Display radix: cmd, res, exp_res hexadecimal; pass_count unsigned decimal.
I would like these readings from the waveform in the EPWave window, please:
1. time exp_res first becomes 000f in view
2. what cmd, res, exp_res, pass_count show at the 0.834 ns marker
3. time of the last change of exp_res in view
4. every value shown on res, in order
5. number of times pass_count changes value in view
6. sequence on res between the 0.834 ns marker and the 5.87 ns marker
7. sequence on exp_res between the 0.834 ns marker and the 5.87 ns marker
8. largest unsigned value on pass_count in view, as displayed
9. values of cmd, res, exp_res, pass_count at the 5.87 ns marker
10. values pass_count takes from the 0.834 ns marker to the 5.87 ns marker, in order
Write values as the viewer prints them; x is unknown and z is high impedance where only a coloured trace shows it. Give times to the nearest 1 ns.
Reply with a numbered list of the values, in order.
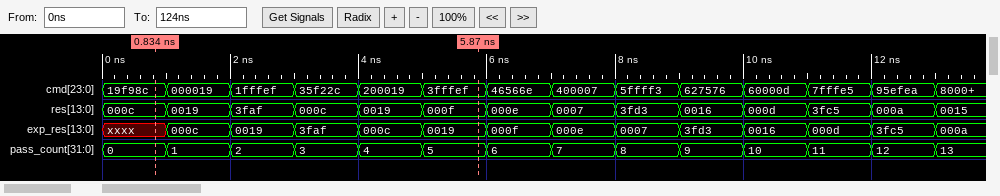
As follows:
1. 6 ns
2. cmd=19f98c, res=000c, exp_res=xxxx, pass_count=0
3. 13 ns
4. 000c, 0019, 3faf, 000c, 0019, 000f, 000e, 0007, 3fd3, 0016, 000d, 3fc5, 000a, 0015
5. 13
6. 000c, 0019, 3faf, 000c, 0019, 000f
7. xxxx, 000c, 0019, 3faf, 000c, 0019
8. 13
9. cmd=3fffef, res=000f, exp_res=0019, pass_count=5
10. 0, 1, 2, 3, 4, 5
